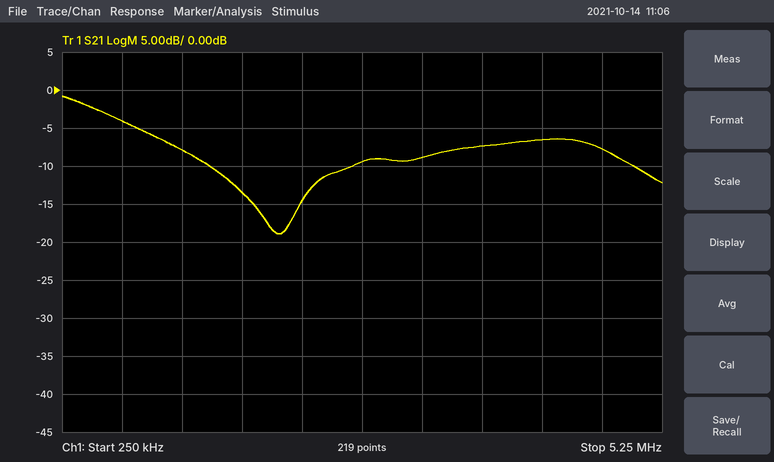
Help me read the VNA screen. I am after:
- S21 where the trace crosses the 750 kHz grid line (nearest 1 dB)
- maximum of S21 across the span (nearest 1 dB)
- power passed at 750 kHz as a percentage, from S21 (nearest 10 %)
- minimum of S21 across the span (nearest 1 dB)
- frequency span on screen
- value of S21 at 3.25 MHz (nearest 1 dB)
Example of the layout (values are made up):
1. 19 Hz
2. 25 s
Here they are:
1. -4 dB
2. -1 dB
3. 40 %
4. -19 dB
5. 5 MHz
6. -9 dB
